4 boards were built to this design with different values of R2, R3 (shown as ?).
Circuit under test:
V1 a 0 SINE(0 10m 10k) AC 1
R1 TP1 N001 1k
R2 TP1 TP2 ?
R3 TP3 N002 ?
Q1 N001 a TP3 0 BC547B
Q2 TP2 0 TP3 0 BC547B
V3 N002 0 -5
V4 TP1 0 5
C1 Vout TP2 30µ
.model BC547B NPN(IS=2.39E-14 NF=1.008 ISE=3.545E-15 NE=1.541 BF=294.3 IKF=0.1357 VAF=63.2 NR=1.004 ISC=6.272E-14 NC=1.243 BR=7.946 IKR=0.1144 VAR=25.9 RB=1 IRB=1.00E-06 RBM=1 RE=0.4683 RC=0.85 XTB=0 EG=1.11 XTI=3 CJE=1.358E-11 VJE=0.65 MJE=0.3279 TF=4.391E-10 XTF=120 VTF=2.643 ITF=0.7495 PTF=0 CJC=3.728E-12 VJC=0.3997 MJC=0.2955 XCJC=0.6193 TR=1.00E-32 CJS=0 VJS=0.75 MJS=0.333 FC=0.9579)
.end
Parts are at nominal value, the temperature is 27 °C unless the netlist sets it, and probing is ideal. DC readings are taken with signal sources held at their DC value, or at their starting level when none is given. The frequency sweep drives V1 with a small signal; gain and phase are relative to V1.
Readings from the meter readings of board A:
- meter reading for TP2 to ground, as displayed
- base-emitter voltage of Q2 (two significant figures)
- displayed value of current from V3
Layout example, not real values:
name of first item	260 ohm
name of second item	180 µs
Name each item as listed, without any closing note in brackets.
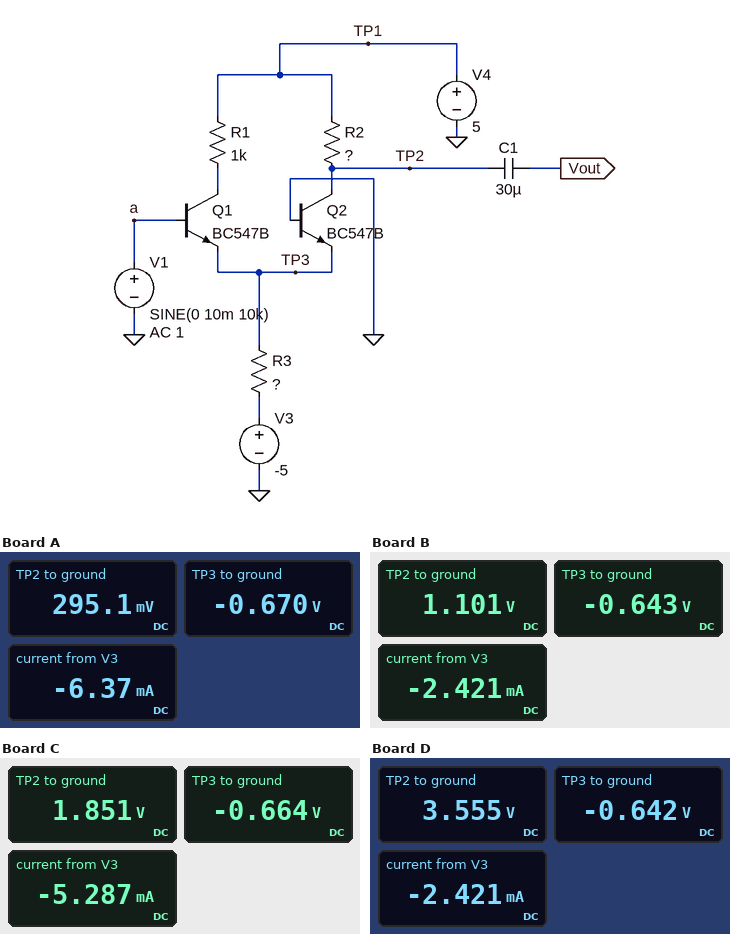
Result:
meter reading for TP2 to ground, as displayed	295.1 mV
base-emitter voltage of Q2	670 mV
displayed value of current from V3	-6.37 mA
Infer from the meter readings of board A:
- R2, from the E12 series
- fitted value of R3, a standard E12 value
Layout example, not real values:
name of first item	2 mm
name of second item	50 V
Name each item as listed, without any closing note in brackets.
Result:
R2, from the E12 series	1.5 kΩ
fitted value of R3, a standard E12 value	680 Ω
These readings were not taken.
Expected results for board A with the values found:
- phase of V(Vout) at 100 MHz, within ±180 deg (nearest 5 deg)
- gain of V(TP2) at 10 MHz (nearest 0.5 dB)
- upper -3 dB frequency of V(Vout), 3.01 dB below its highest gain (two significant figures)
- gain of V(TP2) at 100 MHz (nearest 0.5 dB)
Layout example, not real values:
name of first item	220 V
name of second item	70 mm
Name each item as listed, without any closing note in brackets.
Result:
phase of V(Vout) at 100 MHz, within ±180 deg	-75 deg
gain of V(TP2) at 10 MHz	37.5 dB
upper -3 dB frequency of V(Vout), 3.01 dB below its highest gain	33 MHz
gain of V(TP2) at 100 MHz	28.0 dB
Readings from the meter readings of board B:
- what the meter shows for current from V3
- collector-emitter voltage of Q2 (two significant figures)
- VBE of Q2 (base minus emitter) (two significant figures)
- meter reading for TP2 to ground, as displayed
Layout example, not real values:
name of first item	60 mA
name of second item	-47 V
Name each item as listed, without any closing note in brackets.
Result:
what the meter shows for current from V3	-2.421 mA
collector-emitter voltage of Q2	1.7 V
VBE of Q2 (base minus emitter)	640 mV
meter reading for TP2 to ground, as displayed	1.101 V
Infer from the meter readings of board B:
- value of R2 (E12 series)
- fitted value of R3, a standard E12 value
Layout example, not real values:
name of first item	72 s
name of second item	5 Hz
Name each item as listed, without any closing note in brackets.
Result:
value of R2	3.3 kΩ
fitted value of R3, a standard E12 value	1.8 kΩ
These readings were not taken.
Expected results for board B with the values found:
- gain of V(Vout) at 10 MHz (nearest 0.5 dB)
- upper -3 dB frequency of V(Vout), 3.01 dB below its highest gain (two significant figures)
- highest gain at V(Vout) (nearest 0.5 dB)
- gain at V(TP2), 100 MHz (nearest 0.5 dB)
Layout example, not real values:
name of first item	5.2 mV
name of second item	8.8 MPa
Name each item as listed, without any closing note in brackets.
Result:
gain of V(Vout) at 10 MHz	36.0 dB
upper -3 dB frequency of V(Vout), 3.01 dB below its highest gain	19 MHz
highest gain at V(Vout)	37.0 dB
gain at V(TP2), 100 MHz	22.5 dB
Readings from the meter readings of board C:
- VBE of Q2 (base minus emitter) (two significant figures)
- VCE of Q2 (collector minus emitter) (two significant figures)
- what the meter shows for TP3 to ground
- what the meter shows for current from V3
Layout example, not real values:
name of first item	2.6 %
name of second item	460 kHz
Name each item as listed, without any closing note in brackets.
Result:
VBE of Q2 (base minus emitter)	660 mV
VCE of Q2 (collector minus emitter)	2.5 V
what the meter shows for TP3 to ground	-0.664 V
what the meter shows for current from V3	-5.287 mA
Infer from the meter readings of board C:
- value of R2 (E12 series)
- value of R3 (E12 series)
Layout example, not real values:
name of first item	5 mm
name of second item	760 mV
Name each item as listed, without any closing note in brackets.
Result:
value of R2	1.2 kΩ
value of R3	820 Ω
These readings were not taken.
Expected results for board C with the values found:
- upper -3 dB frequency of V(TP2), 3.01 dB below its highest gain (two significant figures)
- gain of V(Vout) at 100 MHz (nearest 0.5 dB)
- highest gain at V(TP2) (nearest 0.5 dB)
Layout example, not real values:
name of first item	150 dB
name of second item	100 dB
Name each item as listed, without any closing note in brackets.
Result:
upper -3 dB frequency of V(TP2), 3.01 dB below its highest gain	58 MHz
gain of V(Vout) at 100 MHz	28.5 dB
highest gain at V(TP2)	34.5 dB
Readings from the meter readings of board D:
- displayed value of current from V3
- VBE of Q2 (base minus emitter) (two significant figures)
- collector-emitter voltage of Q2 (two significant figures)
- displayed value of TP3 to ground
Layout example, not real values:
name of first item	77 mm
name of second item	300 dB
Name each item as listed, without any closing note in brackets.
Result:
displayed value of current from V3	-2.421 mA
VBE of Q2 (base minus emitter)	640 mV
collector-emitter voltage of Q2	4.2 V
displayed value of TP3 to ground	-0.642 V
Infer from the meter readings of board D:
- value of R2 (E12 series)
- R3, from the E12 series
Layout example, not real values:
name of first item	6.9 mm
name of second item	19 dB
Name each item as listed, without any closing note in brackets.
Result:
value of R2	1.2 kΩ
R3, from the E12 series	1.8 kΩ
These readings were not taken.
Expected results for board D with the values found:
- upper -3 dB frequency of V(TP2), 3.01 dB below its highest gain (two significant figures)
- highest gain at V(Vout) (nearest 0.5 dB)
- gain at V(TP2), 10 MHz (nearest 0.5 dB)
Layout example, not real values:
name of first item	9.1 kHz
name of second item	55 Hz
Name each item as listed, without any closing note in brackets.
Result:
upper -3 dB frequency of V(TP2), 3.01 dB below its highest gain	69 MHz
highest gain at V(Vout)	28.5 dB
gain at V(TP2), 10 MHz	28.5 dB
